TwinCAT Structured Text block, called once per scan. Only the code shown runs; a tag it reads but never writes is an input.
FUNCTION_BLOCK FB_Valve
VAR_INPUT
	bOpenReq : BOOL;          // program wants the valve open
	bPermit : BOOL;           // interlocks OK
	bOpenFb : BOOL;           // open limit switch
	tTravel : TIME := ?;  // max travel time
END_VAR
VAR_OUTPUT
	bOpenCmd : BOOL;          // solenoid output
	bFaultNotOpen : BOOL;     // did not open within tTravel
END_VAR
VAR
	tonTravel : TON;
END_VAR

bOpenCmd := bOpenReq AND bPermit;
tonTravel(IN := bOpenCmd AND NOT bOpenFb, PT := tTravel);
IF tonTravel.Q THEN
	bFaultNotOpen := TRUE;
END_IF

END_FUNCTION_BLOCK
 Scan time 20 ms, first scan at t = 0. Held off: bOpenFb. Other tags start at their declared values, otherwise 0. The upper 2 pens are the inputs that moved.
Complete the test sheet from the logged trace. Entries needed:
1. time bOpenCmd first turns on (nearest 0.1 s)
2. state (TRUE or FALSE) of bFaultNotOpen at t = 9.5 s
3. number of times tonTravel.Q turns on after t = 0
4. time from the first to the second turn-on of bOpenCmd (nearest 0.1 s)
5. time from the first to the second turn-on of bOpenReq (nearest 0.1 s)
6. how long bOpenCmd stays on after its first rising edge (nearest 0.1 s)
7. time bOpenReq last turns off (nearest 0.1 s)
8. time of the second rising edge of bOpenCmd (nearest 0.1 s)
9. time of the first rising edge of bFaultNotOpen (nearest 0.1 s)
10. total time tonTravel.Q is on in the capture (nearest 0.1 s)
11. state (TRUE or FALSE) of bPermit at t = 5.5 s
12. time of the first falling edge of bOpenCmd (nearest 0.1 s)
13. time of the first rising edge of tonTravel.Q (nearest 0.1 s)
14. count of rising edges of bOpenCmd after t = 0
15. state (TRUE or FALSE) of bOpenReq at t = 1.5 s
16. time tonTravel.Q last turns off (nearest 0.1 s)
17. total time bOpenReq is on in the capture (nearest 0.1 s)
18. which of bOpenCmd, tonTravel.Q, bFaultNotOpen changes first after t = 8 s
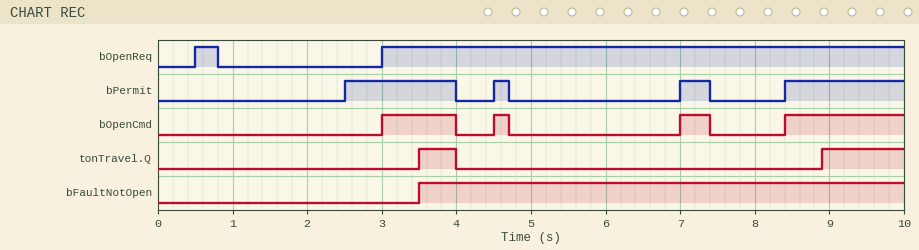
3.0 s
TRUE
2
1.5 s
2.5 s
1.0 s
0.8 s
4.5 s
3.5 s
1.6 s
FALSE
4.0 s
3.5 s
4
FALSE
4.0 s
7.3 s
bOpenCmd
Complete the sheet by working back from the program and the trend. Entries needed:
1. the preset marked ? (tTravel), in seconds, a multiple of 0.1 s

0.5 s
